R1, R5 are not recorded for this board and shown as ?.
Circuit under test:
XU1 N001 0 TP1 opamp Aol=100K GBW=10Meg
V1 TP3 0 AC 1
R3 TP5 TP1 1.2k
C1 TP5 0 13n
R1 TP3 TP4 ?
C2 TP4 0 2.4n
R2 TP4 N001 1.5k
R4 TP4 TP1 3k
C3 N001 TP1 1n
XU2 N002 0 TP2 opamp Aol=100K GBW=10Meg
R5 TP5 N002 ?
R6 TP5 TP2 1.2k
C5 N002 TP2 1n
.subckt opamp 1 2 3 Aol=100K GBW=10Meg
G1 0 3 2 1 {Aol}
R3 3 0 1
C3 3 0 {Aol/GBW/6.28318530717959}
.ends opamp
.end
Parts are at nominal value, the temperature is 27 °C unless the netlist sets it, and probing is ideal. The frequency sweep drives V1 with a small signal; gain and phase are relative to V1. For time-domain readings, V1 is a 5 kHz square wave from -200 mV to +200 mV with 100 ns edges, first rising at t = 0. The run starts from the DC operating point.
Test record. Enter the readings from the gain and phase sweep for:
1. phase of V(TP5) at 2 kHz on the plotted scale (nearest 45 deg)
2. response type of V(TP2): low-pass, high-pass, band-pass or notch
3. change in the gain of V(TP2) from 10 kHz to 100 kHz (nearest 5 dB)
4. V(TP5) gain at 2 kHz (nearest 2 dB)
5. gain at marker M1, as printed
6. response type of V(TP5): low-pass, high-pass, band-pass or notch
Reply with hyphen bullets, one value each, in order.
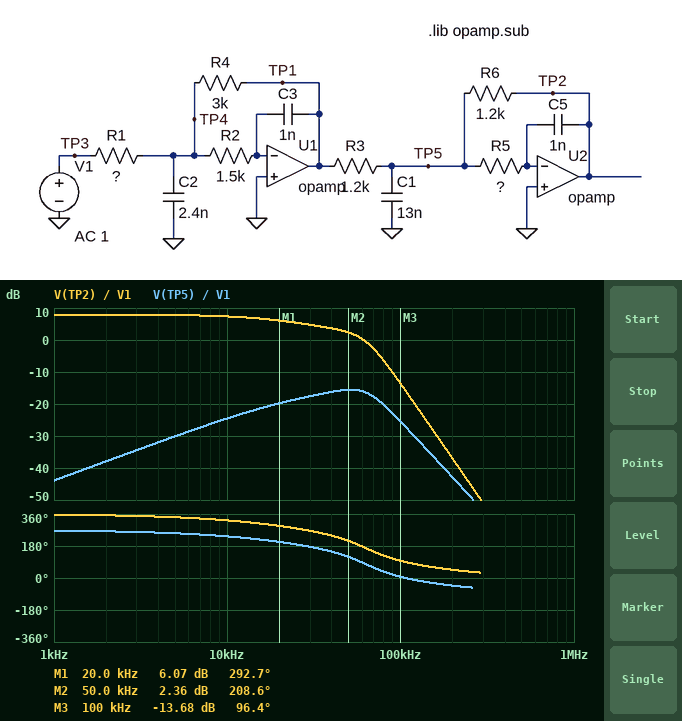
- 270 deg
- low-pass
- -20 dB
- -38 dB
- 6.07 dB
- band-pass
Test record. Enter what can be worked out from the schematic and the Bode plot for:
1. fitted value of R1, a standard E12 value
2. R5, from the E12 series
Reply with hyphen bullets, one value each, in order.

- 1.2 kΩ
- 390 Ω
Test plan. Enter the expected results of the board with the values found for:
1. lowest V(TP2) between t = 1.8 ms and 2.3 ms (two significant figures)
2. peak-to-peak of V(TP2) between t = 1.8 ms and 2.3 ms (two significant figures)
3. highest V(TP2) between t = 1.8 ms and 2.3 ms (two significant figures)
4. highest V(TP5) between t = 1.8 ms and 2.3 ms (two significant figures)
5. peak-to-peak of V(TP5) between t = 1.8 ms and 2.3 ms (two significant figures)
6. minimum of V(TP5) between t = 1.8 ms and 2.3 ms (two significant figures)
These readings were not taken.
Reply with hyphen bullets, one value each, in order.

- -500 mV
- 1.0 V
- 500 mV
- 42 mV
- 83 mV
- -42 mV
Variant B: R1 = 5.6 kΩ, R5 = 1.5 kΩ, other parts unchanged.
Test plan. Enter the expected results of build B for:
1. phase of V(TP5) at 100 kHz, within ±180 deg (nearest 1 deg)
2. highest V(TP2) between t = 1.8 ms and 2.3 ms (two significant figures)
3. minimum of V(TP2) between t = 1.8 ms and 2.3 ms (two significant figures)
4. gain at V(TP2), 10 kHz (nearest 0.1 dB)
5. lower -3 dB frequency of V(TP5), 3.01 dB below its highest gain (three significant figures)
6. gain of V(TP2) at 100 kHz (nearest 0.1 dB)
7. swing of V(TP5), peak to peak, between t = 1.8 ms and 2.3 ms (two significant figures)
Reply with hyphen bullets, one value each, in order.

- -28 deg
- 150 mV
- -150 mV
- -5.0 dB
- 19.5 kHz
- -37.7 dB
- 63 mV
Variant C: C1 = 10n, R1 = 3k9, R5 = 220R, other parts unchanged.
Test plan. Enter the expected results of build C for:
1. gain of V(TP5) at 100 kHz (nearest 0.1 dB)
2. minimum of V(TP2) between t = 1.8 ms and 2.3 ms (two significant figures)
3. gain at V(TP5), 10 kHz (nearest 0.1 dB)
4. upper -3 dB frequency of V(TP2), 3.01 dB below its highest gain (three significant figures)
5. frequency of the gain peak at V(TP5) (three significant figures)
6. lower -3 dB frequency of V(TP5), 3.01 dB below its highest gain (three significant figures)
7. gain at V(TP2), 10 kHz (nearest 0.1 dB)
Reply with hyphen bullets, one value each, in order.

- -33.0 dB
- -160 mV
- -39.0 dB
- 43.3 kHz
- 54.2 kHz
- 24.9 kHz
- -2.4 dB
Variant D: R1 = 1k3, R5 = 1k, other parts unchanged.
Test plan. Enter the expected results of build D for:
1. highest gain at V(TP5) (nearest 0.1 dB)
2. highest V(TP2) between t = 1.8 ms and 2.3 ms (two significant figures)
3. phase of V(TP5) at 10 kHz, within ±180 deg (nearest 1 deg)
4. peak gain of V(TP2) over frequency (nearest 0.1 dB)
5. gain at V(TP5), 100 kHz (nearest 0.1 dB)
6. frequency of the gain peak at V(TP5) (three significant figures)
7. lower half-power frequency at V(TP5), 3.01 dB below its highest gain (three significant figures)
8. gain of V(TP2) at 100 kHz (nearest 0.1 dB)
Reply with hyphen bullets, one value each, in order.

- -8.4 dB
- 500 mV
- -130 deg
- 7.3 dB
- -27.2 dB
- 34.7 kHz
- 20.3 kHz
- -23.3 dB
